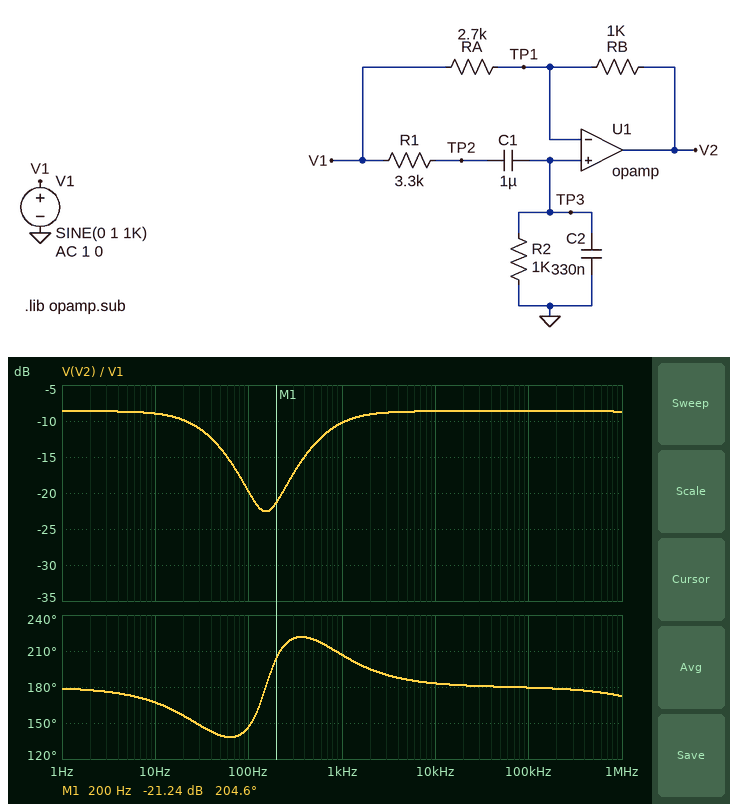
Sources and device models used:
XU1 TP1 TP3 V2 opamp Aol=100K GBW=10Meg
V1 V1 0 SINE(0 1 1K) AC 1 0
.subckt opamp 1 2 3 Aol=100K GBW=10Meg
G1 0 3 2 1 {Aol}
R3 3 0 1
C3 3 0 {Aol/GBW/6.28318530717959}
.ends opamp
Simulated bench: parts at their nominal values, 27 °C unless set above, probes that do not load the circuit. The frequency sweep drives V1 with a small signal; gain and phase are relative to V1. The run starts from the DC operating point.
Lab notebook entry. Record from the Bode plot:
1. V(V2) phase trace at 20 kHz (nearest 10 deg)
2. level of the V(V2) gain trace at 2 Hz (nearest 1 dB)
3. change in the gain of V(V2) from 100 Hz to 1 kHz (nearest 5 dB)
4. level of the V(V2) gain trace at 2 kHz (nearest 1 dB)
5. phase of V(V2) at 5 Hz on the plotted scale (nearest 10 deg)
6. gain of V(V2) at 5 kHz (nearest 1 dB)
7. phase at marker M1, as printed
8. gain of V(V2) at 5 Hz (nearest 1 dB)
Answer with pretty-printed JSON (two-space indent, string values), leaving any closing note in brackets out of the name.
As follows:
{
  "V(V2) phase trace at 20 kHz": "180 deg",
  "level of the V(V2) gain trace at 2 Hz": "-9 dB",
  "change in the gain of V(V2) from 100 Hz to 1 kHz": "10 dB",
  "level of the V(V2) gain trace at 2 kHz": "-9 dB",
  "phase of V(V2) at 5 Hz on the plotted scale": "170 deg",
  "gain of V(V2) at 5 kHz": "-9 dB",
  "phase at marker M1, as printed": "204.6 deg",
  "gain of V(V2) at 5 Hz": "-9 dB"
}
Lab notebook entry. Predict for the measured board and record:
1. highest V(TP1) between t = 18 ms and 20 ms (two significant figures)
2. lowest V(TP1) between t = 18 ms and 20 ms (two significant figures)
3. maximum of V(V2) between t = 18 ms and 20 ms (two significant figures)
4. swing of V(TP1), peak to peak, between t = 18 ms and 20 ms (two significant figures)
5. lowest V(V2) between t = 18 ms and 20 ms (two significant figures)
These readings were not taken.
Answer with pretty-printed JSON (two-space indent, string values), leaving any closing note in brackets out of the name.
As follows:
{
  "highest V(TP1) between t = 18 ms and 20 ms": "120 mV",
  "lowest V(TP1) between t = 18 ms and 20 ms": "-120 mV",
  "maximum of V(V2) between t = 18 ms and 20 ms": "310 mV",
  "swing of V(TP1), peak to peak, between t = 18 ms and 20 ms": "250 mV",
  "lowest V(V2) between t = 18 ms and 20 ms": "-310 mV"
}
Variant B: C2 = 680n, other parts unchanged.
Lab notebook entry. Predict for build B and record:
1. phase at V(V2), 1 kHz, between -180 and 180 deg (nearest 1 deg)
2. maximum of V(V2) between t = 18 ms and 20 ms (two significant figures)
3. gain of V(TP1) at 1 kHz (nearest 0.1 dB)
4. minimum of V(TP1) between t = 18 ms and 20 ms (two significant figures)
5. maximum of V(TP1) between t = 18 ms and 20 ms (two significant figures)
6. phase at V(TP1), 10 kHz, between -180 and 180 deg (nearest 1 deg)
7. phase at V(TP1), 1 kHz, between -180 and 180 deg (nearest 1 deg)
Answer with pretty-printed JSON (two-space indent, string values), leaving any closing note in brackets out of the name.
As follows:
{
  "phase at V(V2), 1 kHz, between -180 and 180 deg": "-166 deg",
  "maximum of V(V2) between t = 18 ms and 20 ms": "350 mV",
  "gain of V(TP1) at 1 kHz": "-23.4 dB",
  "minimum of V(TP1) between t = 18 ms and 20 ms": "-68 mV",
  "maximum of V(TP1) between t = 18 ms and 20 ms": "67 mV",
  "phase at V(TP1), 10 kHz, between -180 and 180 deg": "-88 deg",
  "phase at V(TP1), 1 kHz, between -180 and 180 deg": "-70 deg"
}
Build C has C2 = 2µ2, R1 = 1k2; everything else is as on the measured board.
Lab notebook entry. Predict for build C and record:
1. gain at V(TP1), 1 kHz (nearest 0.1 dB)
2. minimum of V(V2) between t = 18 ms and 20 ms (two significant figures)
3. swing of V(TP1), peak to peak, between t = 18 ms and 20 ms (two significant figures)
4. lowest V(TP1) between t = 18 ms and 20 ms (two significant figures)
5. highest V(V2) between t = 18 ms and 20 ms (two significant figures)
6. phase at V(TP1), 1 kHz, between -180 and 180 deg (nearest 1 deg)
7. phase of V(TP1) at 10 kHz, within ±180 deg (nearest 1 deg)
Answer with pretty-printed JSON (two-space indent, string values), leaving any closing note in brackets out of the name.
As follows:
{
  "gain at V(TP1), 1 kHz": "-24.6 dB",
  "minimum of V(V2) between t = 18 ms and 20 ms": "-360 mV",
  "swing of V(TP1), peak to peak, between t = 18 ms and 20 ms": "120 mV",
  "lowest V(TP1) between t = 18 ms and 20 ms": "-59 mV",
  "highest V(V2) between t = 18 ms and 20 ms": "360 mV",
  "phase at V(TP1), 1 kHz, between -180 and 180 deg": "-75 deg",
  "phase of V(TP1) at 10 kHz, within ±180 deg": "-88 deg"
}
